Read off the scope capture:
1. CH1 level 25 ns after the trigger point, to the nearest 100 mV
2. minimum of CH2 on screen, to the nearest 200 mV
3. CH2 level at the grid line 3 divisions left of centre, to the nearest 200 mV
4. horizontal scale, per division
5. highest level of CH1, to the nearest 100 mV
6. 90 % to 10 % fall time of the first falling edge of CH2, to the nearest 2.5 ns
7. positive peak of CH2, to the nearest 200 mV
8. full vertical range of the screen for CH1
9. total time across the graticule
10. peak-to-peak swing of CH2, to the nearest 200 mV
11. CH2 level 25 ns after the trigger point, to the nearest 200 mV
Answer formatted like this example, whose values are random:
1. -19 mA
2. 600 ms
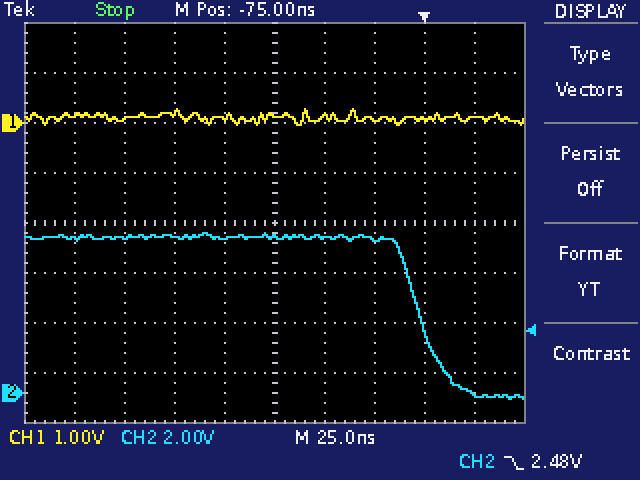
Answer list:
1. 100 mV
2. -200 mV
3. 6.2 V
4. 25 ns
5. 300 mV
6. 25.0 ns
7. 6.4 V
8. 8 V
9. 250 ns
10. 6.6 V
11. 0.0 V
